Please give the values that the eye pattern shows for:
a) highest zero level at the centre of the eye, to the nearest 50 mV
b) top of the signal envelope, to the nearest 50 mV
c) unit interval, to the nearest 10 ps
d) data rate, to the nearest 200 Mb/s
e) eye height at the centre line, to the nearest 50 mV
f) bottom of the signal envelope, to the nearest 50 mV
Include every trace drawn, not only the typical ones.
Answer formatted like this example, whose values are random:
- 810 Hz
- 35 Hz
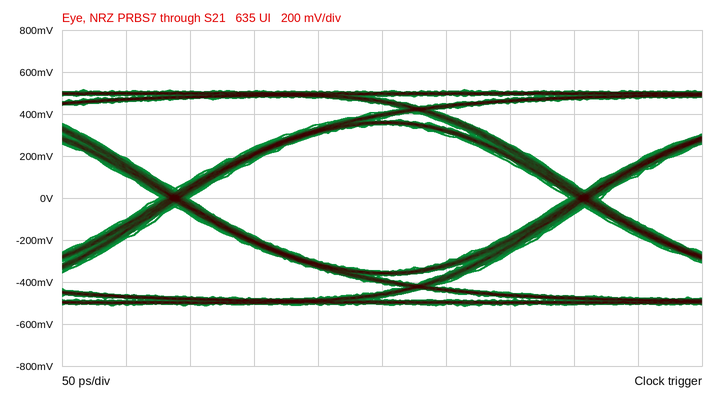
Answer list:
- -350 mV
- 500 mV
- 320 ps
- 3.2 Gb/s
- 700 mV
- -500 mV
